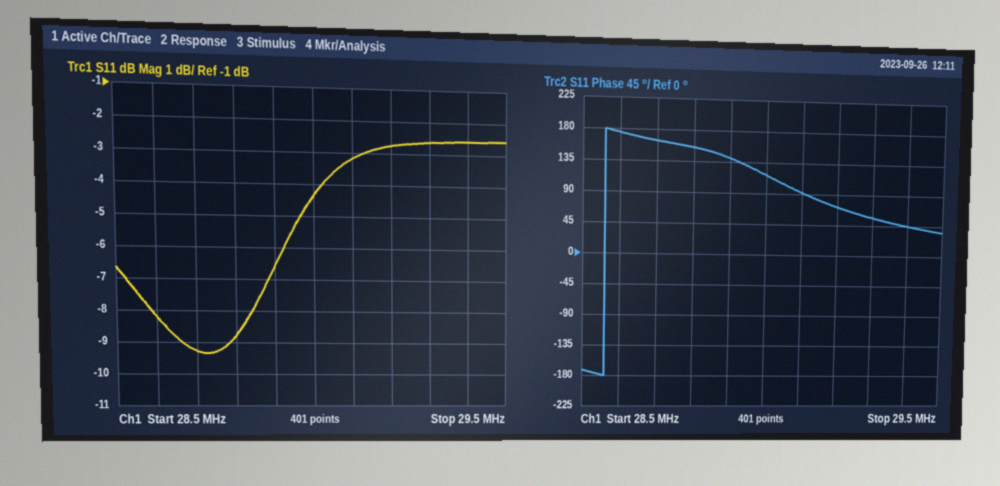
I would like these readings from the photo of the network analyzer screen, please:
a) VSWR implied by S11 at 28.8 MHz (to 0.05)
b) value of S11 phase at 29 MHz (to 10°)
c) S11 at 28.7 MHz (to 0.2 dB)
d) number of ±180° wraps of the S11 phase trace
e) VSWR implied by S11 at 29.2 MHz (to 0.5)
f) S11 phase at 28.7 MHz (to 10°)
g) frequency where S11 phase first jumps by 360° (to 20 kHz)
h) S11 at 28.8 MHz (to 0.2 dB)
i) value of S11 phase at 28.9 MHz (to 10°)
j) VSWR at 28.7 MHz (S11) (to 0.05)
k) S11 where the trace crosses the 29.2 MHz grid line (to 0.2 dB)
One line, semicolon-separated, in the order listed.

2.15; 120°; -9.2 dB; 1; 6.5; 160°; 28.56 MHz; -8.8 dB; 140°; 2.05; -2.8 dB
